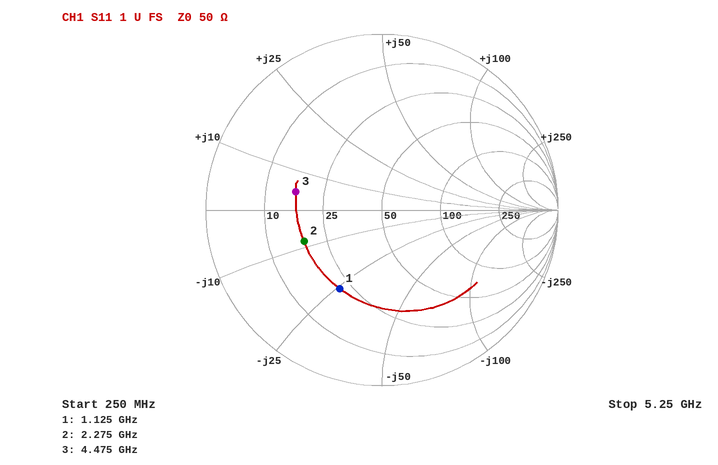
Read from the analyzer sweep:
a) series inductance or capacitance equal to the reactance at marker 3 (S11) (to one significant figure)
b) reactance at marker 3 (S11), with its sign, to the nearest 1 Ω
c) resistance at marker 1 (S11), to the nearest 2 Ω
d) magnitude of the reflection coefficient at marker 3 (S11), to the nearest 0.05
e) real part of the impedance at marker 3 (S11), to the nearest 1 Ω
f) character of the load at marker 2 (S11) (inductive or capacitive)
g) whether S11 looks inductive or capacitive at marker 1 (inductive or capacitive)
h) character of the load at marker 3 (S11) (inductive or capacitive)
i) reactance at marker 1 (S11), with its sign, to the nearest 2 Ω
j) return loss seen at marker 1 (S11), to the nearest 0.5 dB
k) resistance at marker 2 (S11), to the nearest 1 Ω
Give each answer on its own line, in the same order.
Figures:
200 pH
+5 Ω
22 Ω
0.50
17 Ω
capacitive
capacitive
inductive
-26 Ω
6.0 dB
18 Ω
